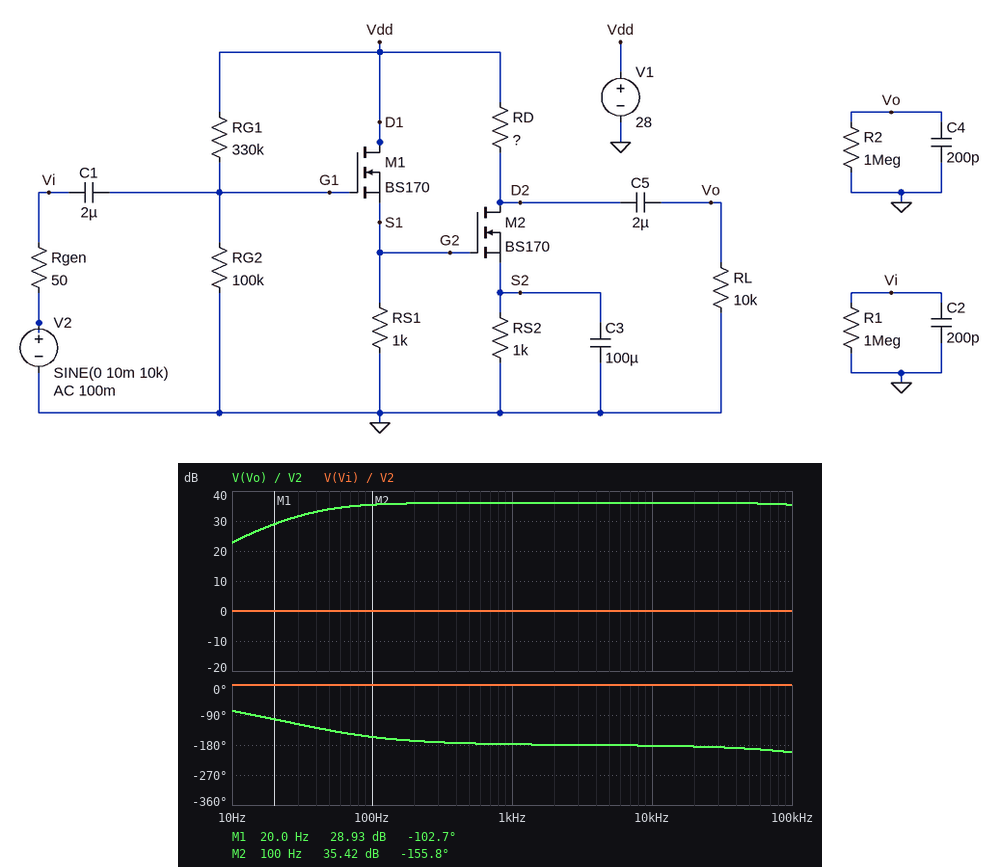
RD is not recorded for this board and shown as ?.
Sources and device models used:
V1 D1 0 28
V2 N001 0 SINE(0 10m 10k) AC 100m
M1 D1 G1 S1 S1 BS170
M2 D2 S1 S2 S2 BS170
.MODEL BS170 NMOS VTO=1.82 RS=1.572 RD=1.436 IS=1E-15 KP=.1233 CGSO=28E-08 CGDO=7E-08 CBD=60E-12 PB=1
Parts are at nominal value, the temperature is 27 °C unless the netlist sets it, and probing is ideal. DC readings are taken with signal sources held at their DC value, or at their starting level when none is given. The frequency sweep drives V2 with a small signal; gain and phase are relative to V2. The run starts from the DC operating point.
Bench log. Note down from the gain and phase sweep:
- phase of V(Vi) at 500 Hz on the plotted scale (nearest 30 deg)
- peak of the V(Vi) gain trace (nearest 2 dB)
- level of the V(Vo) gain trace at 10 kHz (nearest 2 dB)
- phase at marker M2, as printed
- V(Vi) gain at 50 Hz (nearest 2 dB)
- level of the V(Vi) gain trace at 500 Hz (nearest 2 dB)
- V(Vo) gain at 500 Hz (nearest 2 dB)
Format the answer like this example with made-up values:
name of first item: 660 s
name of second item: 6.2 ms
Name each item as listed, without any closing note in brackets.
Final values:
phase of V(Vi) at 500 Hz on the plotted scale: 0 deg
peak of the V(Vi) gain trace: 0 dB
level of the V(Vo) gain trace at 10 kHz: 36 dB
phase at marker M2, as printed: -155.8 deg
V(Vi) gain at 50 Hz: 0 dB
level of the V(Vi) gain trace at 500 Hz: 0 dB
V(Vo) gain at 500 Hz: 36 dB
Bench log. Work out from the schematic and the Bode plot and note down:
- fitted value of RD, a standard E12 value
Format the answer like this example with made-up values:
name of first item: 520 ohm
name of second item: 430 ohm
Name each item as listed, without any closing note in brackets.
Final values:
fitted value of RD, a standard E12 value: 3.9 kΩ
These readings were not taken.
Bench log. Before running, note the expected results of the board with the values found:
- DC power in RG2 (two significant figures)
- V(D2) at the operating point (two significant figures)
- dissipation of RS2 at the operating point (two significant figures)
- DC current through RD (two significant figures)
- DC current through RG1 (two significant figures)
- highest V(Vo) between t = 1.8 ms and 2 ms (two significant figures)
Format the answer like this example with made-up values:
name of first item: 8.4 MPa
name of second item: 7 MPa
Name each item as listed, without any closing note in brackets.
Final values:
DC power in RG2: 420 µW
V(D2) at the operating point: 19 V
dissipation of RS2 at the operating point: 5.7 mW
DC current through RD: 2.4 mA
DC current through RG1: 65 µA
highest V(Vo) between t = 1.8 ms and 2 ms: 620 mV
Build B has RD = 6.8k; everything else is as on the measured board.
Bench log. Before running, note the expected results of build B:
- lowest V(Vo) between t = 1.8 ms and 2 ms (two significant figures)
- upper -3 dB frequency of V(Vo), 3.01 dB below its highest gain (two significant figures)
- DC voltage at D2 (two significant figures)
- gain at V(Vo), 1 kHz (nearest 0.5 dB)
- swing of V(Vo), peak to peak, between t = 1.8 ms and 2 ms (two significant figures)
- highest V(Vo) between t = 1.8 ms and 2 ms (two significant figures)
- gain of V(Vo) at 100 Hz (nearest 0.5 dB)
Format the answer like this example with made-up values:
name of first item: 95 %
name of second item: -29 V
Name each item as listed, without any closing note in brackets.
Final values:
lowest V(Vo) between t = 1.8 ms and 2 ms: -930 mV
upper -3 dB frequency of V(Vo), 3.01 dB below its highest gain: 170 kHz
DC voltage at D2: 12 V
gain at V(Vo), 1 kHz: 39.0 dB
swing of V(Vo), peak to peak, between t = 1.8 ms and 2 ms: 1.8 V
highest V(Vo) between t = 1.8 ms and 2 ms: 900 mV
gain of V(Vo) at 100 Hz: 38.5 dB
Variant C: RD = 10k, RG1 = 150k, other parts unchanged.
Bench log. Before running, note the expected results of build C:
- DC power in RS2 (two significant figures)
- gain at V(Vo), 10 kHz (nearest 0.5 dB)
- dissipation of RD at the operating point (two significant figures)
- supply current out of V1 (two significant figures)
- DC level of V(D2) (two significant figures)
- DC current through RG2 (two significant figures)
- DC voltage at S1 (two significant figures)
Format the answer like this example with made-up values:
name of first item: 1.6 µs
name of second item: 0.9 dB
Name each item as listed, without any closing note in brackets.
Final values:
DC power in RS2: 6.5 mW
gain at V(Vo), 10 kHz: -60.5 dB
dissipation of RD at the operating point: 65 mW
supply current out of V1: 12 mA
DC level of V(D2): 2.6 V
DC current through RG2: 110 µA
DC voltage at S1: 9.0 V
